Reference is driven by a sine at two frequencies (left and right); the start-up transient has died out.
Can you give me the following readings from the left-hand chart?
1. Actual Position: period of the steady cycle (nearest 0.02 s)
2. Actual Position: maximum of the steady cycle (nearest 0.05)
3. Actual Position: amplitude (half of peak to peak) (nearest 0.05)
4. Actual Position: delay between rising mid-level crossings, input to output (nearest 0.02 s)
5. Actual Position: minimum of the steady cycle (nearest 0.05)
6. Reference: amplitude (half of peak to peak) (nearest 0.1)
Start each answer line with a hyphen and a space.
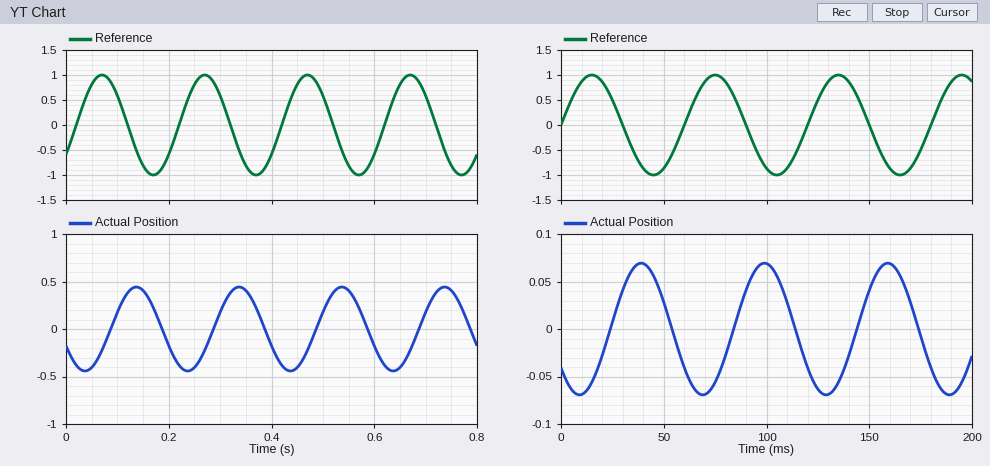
- 0.20 s
- 0.45
- 0.45
- 0.06 s
- -0.45
- 1.0
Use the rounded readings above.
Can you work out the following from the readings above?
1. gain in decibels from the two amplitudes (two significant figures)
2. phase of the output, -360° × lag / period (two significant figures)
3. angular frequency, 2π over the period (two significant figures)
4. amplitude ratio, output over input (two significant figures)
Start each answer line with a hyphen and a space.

- -6.9 dB
- -110°
- 31 rad/s
- 0.45
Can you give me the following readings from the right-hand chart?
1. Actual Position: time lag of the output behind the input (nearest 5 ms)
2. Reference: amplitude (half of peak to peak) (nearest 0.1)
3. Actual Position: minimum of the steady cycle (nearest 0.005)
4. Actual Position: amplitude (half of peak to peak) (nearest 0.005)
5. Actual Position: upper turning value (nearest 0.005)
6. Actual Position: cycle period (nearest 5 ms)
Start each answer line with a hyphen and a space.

- 25 ms
- 1.0
- -0.070
- 0.070
- 0.070
- 60 ms
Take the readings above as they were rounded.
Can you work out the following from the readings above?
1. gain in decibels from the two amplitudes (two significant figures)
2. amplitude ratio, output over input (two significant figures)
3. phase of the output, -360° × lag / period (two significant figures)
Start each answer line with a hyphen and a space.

- -23 dB
- 0.070
- -150°
